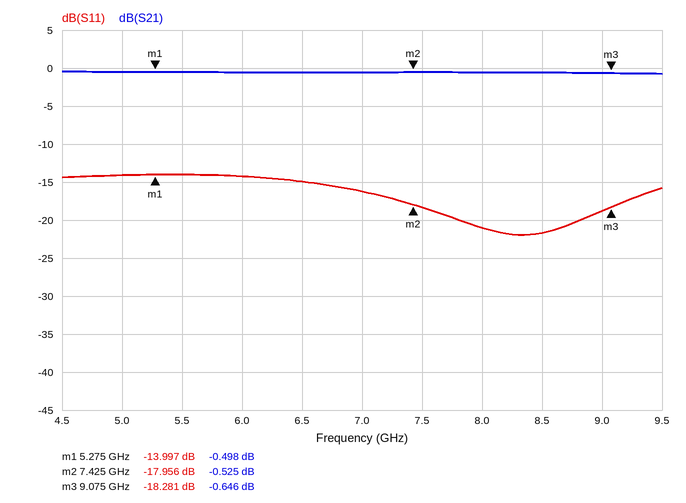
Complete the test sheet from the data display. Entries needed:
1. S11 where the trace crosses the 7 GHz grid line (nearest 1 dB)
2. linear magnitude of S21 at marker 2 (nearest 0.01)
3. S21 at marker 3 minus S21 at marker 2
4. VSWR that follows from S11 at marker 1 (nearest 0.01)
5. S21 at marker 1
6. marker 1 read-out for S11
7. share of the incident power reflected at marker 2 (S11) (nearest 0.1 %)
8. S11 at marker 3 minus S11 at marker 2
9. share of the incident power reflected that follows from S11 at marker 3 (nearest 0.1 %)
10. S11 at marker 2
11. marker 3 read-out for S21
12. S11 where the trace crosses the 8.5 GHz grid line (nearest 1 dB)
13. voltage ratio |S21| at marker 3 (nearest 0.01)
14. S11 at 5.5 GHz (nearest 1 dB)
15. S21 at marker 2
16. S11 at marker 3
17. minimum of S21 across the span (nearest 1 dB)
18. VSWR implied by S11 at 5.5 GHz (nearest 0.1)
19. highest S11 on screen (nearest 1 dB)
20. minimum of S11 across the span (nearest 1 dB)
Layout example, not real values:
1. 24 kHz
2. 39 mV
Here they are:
1. -16 dB
2. 0.94
3. -0.121 dB
4. 1.50
5. -0.498 dB
6. -13.997 dB
7. 1.6 %
8. -0.325 dB
9. 1.5 %
10. -17.956 dB
11. -0.646 dB
12. -22 dB
13. 0.93
14. -14 dB
15. -0.525 dB
16. -18.281 dB
17. -1 dB
18. 1.5
19. -14 dB
20. -22 dB
